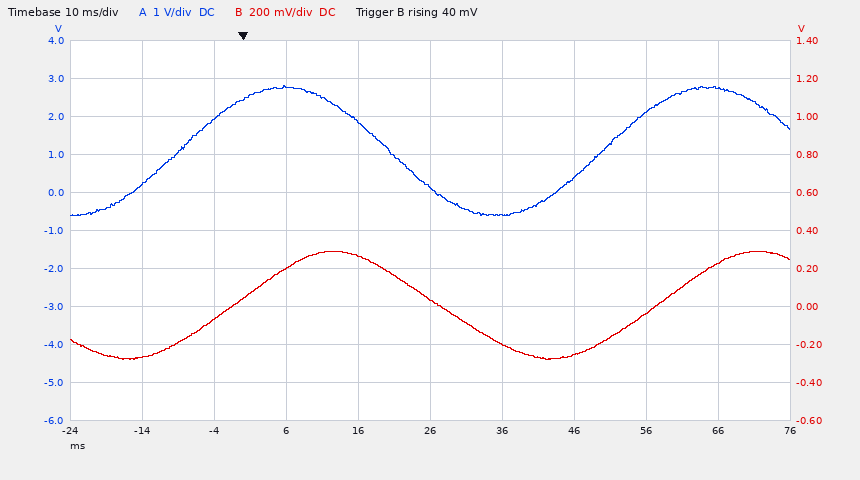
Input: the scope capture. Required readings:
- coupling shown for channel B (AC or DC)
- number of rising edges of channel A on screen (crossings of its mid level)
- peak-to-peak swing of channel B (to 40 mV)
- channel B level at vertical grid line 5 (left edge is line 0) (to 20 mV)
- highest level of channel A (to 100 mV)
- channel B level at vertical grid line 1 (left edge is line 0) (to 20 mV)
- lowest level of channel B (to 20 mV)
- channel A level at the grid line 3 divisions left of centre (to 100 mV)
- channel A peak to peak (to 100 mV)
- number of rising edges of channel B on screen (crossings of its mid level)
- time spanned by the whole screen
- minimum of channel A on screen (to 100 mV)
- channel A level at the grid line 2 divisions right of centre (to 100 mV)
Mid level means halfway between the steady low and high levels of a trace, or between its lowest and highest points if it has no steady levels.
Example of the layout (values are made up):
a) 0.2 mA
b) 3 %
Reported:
a) DC
b) 2
c) 560 mV
d) 40 mV
e) 2.8 V
f) -260 mV
g) -280 mV
h) 1.9 V
i) 3.4 V
j) 2
k) 100 ms
l) -600 mV
m) 400 mV
